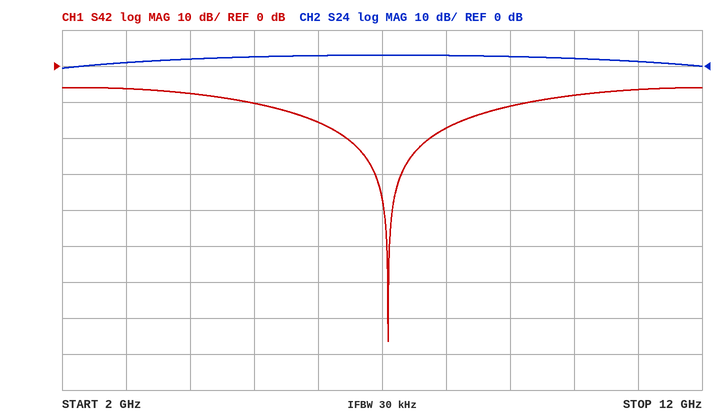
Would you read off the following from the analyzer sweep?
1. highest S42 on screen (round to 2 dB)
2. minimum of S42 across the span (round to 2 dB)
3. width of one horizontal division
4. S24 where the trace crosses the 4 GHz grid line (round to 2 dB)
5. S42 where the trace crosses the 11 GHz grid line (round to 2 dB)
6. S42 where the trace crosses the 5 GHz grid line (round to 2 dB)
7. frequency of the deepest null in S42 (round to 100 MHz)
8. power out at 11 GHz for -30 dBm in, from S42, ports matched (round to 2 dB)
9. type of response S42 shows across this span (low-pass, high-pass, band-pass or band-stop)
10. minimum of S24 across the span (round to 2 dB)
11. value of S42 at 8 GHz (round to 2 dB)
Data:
-6 dB
-76 dB
1 GHz
2 dB
-6 dB
-10 dB
7.1 GHz
-36 dBm
band-stop
0 dB
-18 dB
